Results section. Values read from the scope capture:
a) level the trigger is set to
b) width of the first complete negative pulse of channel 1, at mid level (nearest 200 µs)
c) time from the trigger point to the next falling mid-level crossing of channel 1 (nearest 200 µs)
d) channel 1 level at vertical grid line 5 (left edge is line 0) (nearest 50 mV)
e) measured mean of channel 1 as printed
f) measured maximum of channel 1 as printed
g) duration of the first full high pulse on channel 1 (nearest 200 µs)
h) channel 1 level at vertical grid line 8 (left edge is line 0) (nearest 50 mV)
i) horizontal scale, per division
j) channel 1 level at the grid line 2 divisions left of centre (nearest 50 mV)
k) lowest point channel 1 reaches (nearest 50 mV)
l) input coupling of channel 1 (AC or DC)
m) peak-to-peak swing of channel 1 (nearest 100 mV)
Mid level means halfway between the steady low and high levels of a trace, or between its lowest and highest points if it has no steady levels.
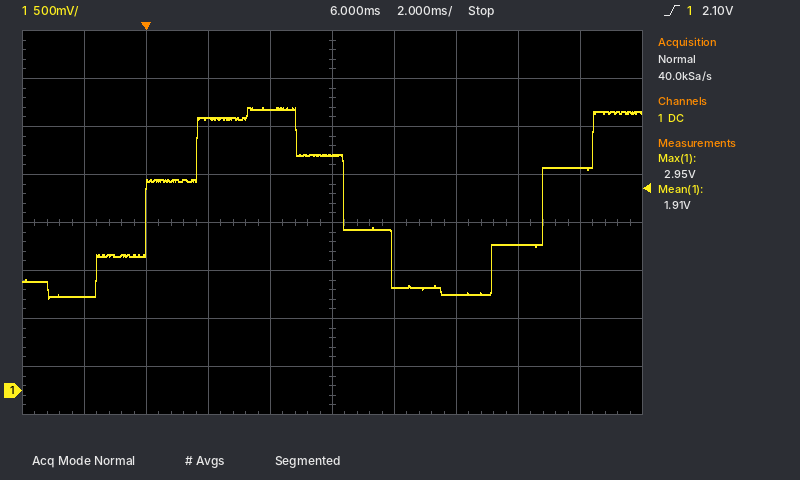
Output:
2.10 V
6.4 ms
6.4 ms
2.45 V
1.91 V
2.95 V
6.4 ms
1.50 V
2 ms
2.85 V
950 mV
DC
2.00 V
